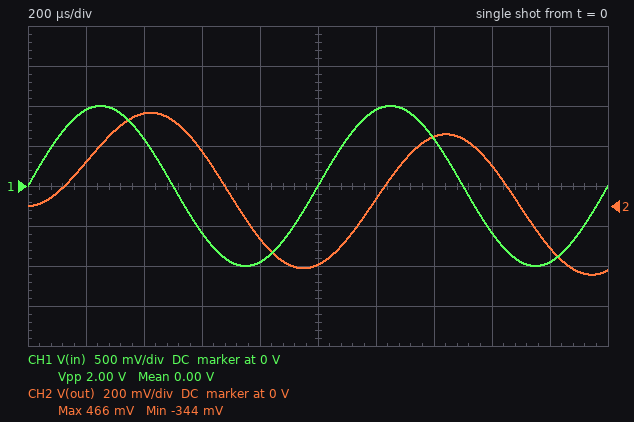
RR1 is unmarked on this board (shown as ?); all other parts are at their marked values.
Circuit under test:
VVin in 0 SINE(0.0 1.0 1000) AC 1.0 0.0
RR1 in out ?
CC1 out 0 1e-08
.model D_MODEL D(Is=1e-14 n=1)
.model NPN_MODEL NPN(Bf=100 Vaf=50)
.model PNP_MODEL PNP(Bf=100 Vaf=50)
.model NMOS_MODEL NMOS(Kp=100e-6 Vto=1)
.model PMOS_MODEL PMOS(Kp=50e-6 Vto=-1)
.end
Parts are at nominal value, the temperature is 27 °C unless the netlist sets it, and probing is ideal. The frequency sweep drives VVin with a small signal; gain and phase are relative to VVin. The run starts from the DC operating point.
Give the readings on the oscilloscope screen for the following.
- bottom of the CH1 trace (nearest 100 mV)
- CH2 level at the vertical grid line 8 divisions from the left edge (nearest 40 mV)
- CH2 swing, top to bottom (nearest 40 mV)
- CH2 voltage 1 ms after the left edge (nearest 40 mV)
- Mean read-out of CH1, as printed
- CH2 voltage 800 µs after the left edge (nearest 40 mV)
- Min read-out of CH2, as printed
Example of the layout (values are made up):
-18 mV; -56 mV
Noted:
-1.0 V; 200 mV; 800 mV; -280 mV; 0.00 V; -160 mV; -344 mV
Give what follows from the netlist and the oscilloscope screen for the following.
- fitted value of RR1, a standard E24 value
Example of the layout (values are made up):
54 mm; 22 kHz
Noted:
43 kΩ
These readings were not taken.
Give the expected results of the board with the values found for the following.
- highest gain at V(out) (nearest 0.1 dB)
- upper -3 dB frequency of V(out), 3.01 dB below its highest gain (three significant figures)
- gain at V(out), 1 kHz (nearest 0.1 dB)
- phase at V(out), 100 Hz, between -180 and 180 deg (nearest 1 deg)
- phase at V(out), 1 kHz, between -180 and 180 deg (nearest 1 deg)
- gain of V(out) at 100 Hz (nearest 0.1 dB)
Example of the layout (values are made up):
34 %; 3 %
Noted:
0 dB; 370 Hz; -9.2 dB; -15 deg; -70 deg; -0.3 dB
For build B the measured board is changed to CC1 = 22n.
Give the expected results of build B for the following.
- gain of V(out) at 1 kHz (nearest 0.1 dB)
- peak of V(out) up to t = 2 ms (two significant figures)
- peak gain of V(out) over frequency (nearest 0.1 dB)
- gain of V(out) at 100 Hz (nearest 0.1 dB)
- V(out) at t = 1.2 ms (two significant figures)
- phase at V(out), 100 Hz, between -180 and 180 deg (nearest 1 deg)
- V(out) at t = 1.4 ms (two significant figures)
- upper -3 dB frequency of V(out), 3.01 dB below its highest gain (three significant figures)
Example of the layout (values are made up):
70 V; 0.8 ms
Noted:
-15.6 dB; 270 mV; 0 dB; -1.3 dB; 22 mV; -31 deg; 190 mV; 168 Hz
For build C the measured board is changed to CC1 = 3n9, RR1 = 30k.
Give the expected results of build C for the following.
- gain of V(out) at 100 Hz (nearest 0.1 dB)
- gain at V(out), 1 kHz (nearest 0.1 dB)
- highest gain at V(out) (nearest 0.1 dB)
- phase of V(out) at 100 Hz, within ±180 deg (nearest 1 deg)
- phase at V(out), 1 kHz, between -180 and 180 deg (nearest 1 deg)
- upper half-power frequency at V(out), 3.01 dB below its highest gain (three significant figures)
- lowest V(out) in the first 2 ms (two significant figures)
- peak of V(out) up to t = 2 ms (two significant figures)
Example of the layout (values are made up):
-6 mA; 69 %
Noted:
0 dB; -1.9 dB; 0 dB; -4 deg; -36 deg; 1.36 kHz; -810 mV; 830 mV
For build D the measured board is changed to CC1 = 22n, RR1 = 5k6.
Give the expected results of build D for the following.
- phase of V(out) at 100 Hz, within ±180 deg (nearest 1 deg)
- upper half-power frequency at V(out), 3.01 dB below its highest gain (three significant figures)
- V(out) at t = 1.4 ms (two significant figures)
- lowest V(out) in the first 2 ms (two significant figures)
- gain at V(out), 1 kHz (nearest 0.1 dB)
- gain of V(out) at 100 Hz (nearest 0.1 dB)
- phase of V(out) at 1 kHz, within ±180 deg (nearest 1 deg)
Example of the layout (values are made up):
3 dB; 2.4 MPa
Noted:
-4 deg; 1.29 kHz; 760 mV; -790 mV; -2.0 dB; 0 dB; -38 deg
